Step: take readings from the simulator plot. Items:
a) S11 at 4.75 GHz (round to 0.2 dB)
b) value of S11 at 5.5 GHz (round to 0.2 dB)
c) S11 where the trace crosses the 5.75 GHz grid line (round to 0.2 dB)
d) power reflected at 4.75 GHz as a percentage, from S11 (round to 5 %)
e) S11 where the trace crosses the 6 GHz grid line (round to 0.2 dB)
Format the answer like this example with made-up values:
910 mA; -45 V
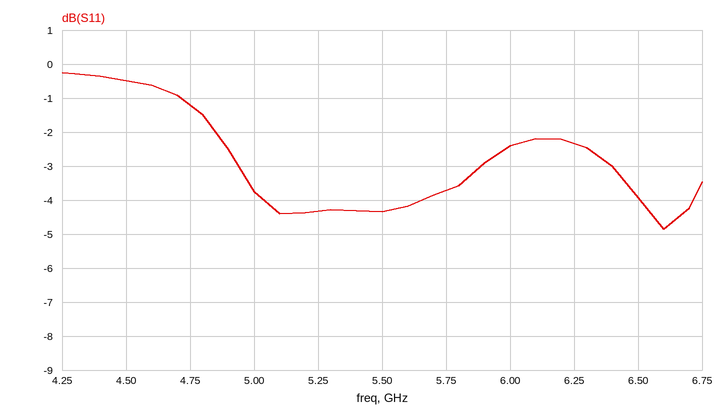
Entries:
-1.2 dB; -4.4 dB; -3.8 dB; 75 %; -2.4 dB
